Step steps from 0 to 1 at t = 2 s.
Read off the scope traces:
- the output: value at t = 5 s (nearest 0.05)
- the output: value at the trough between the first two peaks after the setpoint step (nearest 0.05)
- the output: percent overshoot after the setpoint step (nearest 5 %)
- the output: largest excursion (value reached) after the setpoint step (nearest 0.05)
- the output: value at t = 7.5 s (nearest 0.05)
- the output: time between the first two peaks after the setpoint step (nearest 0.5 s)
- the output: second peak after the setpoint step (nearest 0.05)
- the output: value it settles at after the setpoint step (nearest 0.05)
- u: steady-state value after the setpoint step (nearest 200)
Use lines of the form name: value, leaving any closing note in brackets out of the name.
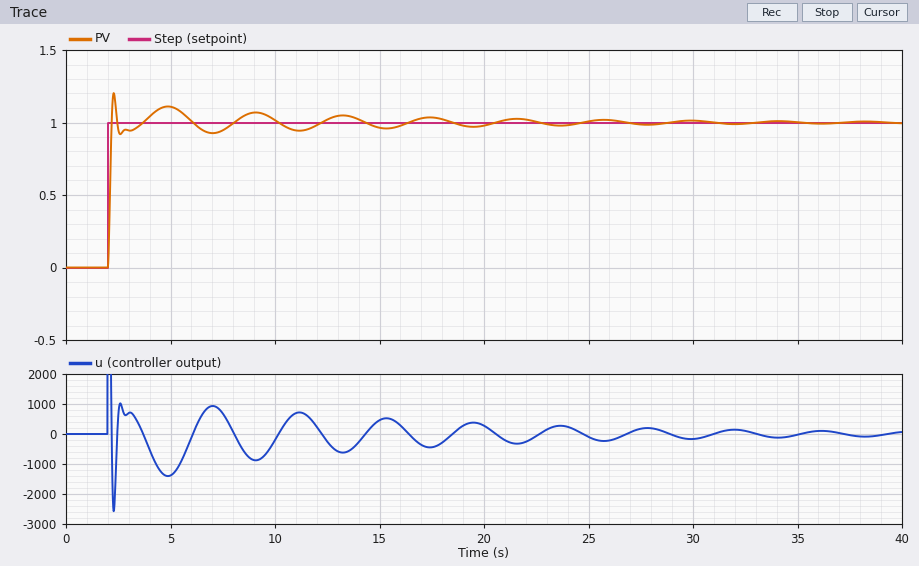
the output: value at t = 5 s: 1.10
the output: value at the trough between the first two peaks after the setpoint step: 0.90
the output: percent overshoot after the setpoint step: 20 %
the output: largest excursion (value reached) after the setpoint step: 1.20
the output: value at t = 7.5 s: 0.95
the output: time between the first two peaks after the setpoint step: 2.5 s
the output: second peak after the setpoint step: 1.10
the output: value it settles at after the setpoint step: 1.00
u: steady-state value after the setpoint step: 0
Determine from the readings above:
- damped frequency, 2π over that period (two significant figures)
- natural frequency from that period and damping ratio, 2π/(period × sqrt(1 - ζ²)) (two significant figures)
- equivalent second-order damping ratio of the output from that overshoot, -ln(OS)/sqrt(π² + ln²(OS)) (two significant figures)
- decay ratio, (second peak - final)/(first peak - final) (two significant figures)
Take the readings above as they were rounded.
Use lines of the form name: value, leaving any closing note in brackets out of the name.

damped frequency, 2π over that period: 2.5 rad/s
natural frequency from that period and damping ratio, 2π/(period × sqrt(1 - ζ²)): 2.8 rad/s
equivalent second-order damping ratio of the output from that overshoot, -ln(OS)/sqrt(π² + ln²(OS)): 0.46
decay ratio, (second peak - final)/(first peak - final): 0.50
